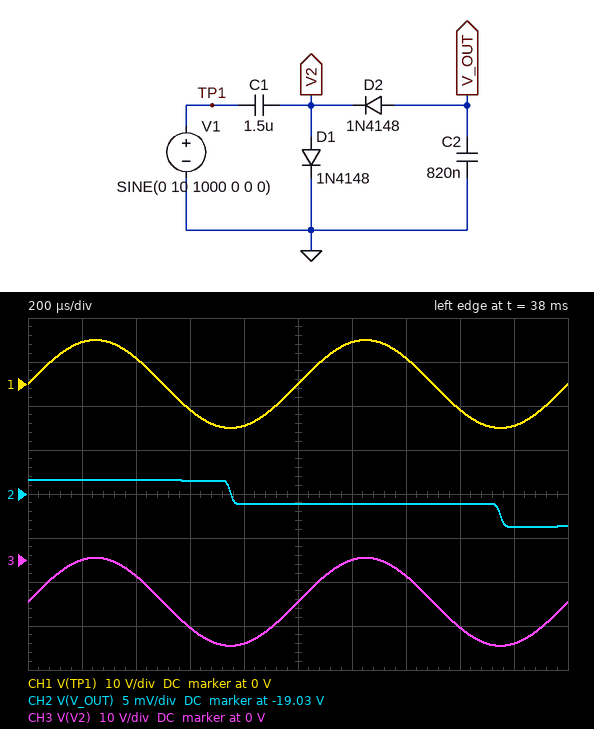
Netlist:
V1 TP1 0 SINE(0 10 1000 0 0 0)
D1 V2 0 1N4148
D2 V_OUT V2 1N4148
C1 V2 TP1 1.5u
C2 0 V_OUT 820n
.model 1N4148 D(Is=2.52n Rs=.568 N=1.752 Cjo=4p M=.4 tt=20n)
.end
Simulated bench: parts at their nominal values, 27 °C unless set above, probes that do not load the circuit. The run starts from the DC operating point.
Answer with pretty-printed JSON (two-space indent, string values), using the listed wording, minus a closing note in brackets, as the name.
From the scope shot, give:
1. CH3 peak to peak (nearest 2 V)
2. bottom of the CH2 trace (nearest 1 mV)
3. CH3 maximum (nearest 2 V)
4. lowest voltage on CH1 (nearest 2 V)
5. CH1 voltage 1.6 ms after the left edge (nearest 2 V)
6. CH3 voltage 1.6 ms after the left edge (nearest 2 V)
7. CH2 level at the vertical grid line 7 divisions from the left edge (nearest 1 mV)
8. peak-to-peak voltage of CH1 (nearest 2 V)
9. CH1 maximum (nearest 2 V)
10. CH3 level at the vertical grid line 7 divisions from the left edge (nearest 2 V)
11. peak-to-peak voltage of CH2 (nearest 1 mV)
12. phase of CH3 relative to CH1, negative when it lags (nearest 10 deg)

{
  "CH3 peak to peak": "20 V",
  "bottom of the CH2 trace": "-19.034 V",
  "CH3 maximum": "0 V",
  "lowest voltage on CH1": "-10 V",
  "CH1 voltage 1.6 ms after the left edge": "-6 V",
  "CH3 voltage 1.6 ms after the left edge": "-16 V",
  "CH2 level at the vertical grid line 7 divisions from the left edge": "-19.031 V",
  "peak-to-peak voltage of CH1": "20 V",
  "CH1 maximum": "10 V",
  "CH3 level at the vertical grid line 7 divisions from the left edge": "-4 V",
  "peak-to-peak voltage of CH2": "5 mV",
  "phase of CH3 relative to CH1, negative when it lags": "0 deg"
}
